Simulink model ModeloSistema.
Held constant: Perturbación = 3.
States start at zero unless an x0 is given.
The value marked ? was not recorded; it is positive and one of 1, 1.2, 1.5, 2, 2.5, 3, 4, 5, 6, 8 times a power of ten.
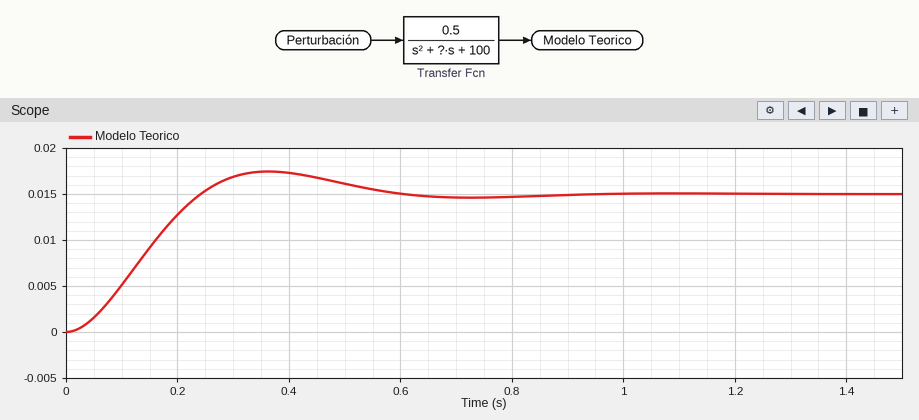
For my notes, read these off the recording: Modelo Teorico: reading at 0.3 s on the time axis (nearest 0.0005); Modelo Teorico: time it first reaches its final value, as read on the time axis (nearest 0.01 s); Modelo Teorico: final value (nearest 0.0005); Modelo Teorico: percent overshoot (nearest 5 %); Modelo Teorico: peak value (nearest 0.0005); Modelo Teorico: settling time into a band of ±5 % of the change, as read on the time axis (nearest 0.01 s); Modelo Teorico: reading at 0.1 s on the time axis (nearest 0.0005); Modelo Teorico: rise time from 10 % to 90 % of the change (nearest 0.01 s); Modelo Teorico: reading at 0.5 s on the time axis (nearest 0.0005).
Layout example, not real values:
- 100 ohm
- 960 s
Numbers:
- 0.0170
- 0.24 s
- 0.0150
- 15 %
- 0.0175
- 0.53 s
- 0.0050
- 0.16 s
- 0.0160
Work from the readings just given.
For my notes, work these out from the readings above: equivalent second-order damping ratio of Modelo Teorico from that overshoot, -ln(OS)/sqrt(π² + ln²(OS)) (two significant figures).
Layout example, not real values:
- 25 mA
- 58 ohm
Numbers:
- 0.52
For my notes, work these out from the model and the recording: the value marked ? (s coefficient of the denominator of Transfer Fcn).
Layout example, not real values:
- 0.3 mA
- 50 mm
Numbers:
- 10
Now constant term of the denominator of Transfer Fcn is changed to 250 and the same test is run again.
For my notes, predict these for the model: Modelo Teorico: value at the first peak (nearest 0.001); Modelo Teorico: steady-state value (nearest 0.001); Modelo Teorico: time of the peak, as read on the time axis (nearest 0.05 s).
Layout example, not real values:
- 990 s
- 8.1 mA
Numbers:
- 0.008
- 0.006
- 0.20 s
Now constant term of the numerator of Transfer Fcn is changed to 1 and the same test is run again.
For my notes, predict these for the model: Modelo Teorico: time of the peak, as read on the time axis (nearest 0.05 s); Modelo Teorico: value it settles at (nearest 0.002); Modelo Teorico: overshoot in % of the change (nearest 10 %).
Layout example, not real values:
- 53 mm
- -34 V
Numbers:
- 0.35 s
- 0.030
- 20 %
